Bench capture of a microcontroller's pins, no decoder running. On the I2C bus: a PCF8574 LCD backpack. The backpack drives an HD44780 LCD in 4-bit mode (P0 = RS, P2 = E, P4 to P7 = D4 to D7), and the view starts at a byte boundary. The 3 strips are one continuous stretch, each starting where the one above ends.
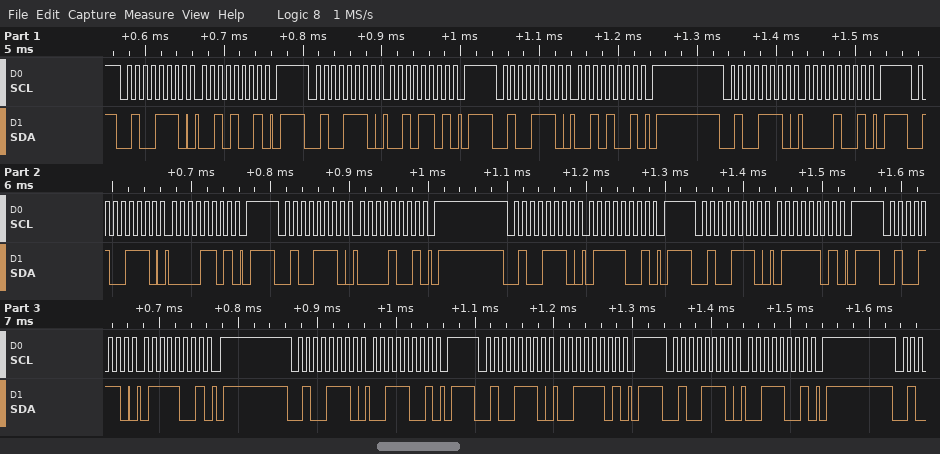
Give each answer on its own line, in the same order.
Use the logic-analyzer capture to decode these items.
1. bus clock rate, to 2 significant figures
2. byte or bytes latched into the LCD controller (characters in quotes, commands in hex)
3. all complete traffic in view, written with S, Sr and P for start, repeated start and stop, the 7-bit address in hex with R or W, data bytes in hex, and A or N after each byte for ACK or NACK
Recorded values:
100 kHz
' ' 's'
S 27W A 29 A P S 27W A 2D A P S 27W A 29 A P S 27W A 09 A P S 27W A 0D A P S 27W A 09 A P S 27W A 79 A P S 27W A 7D A P S 27W A 79 A P S 27W A 39 A P S 27W A 3D A P S 27W A 39 A P
